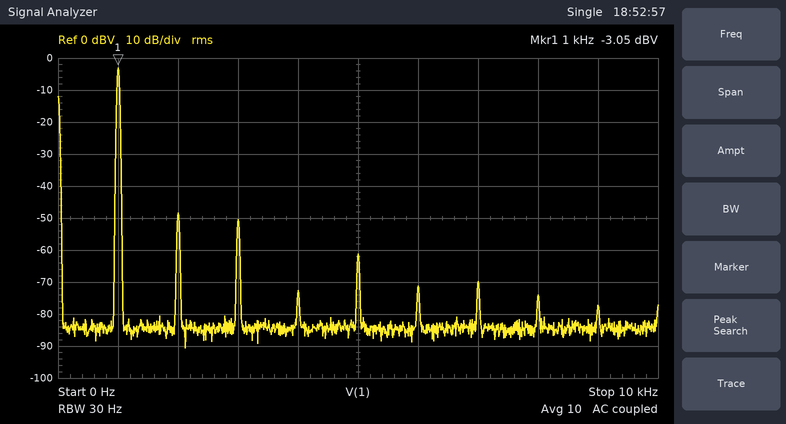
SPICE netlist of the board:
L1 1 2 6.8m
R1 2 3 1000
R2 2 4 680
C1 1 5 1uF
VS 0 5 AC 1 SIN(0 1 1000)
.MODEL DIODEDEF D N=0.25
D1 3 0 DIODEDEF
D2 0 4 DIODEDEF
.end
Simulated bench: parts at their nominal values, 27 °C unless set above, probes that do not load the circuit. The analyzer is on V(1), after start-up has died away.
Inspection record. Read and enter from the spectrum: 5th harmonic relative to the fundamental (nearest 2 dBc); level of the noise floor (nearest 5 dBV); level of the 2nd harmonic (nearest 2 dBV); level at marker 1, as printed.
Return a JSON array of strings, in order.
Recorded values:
["-58 dBc", "-85 dBV", "-48 dBV", "-3.05 dBV"]
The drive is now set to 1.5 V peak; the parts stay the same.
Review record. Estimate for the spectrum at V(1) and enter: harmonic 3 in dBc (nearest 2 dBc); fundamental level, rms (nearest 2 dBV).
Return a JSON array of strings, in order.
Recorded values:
["-50 dBc", "0 dBV"]
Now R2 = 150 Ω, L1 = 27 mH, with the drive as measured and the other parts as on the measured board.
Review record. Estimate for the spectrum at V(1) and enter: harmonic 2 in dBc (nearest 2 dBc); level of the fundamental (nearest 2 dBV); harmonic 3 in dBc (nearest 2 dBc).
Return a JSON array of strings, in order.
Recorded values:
["-30 dBc", "-2 dBV", "-40 dBc"]
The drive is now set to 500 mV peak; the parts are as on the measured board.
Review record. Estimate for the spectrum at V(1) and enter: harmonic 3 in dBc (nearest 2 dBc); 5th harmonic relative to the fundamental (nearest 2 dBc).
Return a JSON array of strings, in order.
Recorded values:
["-44 dBc", "-56 dBc"]
